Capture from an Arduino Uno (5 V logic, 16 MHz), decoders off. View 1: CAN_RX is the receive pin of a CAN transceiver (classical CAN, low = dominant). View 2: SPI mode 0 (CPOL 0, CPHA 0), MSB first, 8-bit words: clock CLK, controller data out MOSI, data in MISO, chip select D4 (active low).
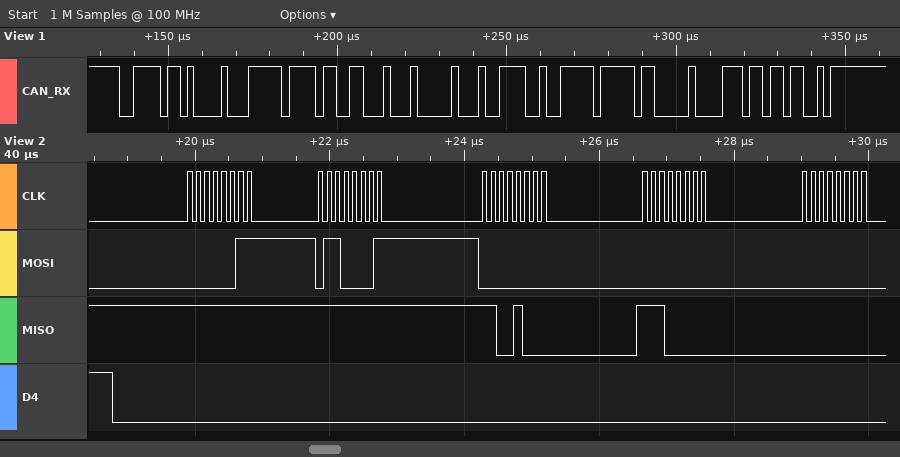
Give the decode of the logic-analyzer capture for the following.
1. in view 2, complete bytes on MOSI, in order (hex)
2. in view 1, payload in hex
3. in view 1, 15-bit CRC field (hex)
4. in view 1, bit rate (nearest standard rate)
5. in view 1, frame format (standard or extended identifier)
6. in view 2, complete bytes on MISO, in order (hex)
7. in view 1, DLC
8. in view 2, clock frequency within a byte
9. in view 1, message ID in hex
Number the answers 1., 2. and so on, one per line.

1. 0x03 0x61 0x00 0x00 0x00
2. FF B3 11 00 9E 4F FF 00
3. 0x3B6C
4. 500 kbit/s
5. standard
6. 0xFF 0xFF 0xC8 0xE0 0x00
7. 8
8. 8 MHz
9. 0x3DA
